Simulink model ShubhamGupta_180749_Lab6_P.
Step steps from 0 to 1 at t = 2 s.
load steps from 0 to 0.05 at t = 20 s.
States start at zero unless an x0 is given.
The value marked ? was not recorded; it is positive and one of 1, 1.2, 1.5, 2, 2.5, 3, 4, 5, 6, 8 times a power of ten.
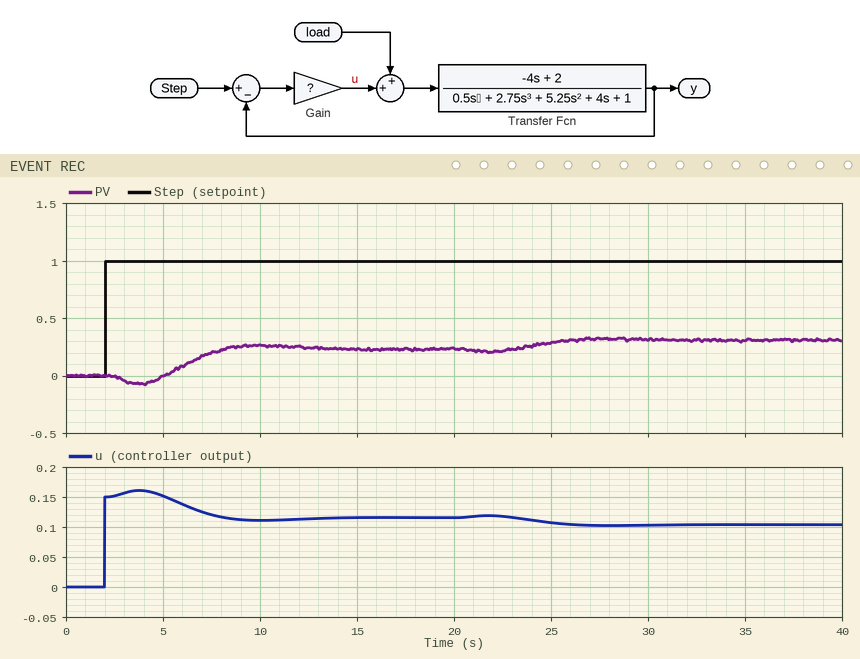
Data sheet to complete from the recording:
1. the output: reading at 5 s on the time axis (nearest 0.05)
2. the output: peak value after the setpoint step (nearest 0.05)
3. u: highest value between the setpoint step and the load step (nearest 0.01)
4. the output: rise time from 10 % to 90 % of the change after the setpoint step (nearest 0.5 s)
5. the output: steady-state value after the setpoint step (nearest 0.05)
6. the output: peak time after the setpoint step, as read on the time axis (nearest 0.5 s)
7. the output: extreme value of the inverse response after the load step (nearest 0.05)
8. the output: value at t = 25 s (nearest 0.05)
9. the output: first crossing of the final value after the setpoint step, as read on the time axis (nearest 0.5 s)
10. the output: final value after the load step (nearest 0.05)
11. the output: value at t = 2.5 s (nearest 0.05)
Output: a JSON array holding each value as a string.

["0.00", "0.25", "0.16", "2.5 s", "0.25", "10.0 s", "0.20", "0.30", "8.0 s", "0.30", "0.00"]
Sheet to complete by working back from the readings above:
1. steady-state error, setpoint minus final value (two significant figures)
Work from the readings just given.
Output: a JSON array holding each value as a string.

["0.75"]
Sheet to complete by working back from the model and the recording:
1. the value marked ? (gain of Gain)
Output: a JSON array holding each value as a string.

["0.15"]
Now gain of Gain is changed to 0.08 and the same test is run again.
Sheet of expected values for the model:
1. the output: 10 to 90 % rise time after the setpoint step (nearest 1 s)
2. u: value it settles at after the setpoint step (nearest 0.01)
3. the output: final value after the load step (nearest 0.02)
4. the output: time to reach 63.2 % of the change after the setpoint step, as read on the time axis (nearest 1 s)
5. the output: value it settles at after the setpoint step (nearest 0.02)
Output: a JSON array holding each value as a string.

["3 s", "0.07", "0.22", "7 s", "0.14"]
